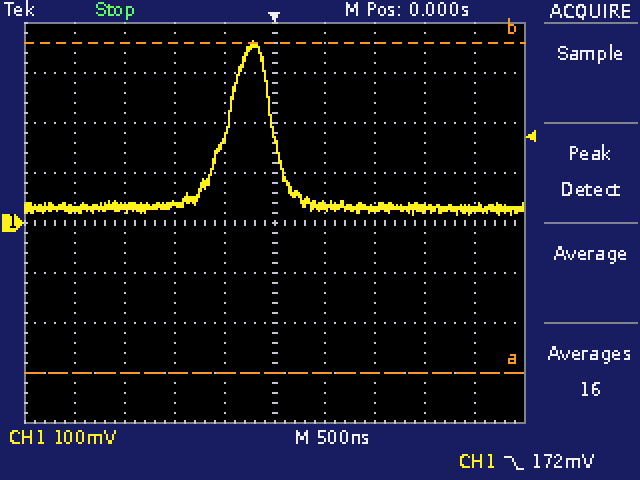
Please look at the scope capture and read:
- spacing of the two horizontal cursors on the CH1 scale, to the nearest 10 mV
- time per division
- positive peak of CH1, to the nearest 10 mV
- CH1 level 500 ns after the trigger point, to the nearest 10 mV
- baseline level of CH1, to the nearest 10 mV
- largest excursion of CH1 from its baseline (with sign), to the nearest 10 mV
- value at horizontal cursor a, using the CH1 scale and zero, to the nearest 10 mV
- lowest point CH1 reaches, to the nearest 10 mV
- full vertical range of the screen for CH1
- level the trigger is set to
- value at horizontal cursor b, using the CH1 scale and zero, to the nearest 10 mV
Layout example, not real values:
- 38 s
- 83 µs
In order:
- 660 mV
- 500 ns
- 360 mV
- 30 mV
- 30 mV
- +330 mV
- -300 mV
- 20 mV
- 800 mV
- 172 mV
- 360 mV
